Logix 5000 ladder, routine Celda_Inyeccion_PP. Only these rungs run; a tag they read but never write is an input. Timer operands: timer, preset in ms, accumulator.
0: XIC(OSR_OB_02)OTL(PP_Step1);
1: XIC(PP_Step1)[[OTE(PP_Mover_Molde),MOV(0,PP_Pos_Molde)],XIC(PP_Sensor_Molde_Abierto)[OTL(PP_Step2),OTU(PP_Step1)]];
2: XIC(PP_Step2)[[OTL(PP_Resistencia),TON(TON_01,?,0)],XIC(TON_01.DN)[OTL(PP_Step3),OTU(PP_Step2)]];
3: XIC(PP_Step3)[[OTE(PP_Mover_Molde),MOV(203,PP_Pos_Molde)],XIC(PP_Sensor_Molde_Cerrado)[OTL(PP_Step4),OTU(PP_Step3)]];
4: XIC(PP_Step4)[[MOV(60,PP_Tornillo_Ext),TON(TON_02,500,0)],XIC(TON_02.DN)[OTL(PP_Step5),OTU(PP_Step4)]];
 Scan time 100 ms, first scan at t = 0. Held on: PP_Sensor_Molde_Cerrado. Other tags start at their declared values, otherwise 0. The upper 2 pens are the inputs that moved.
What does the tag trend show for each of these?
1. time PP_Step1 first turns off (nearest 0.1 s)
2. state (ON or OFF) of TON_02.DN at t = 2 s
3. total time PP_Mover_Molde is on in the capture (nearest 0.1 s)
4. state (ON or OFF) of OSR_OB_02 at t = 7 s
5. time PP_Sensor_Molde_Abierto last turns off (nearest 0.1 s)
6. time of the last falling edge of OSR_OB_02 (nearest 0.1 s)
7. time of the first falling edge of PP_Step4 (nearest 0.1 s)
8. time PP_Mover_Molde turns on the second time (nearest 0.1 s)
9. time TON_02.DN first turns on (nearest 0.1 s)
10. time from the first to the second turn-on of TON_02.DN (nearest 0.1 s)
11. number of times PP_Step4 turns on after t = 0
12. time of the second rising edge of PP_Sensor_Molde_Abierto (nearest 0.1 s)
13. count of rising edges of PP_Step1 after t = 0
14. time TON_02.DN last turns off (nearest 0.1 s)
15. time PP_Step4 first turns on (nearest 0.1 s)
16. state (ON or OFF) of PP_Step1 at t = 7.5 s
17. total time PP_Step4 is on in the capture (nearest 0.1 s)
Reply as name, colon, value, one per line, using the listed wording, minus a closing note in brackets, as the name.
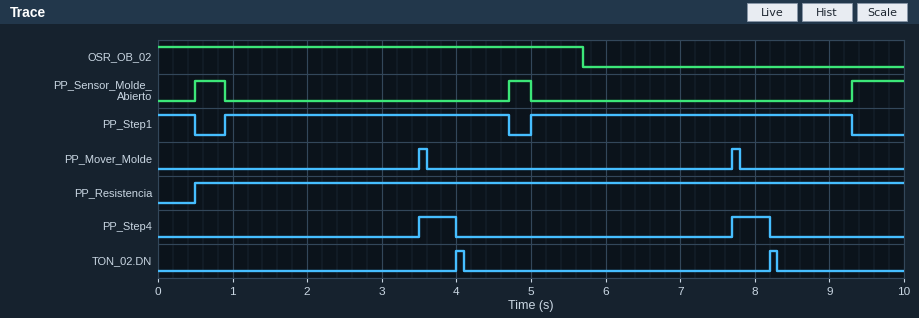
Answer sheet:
time PP_Step1 first turns off: 0.5 s
state (ON or OFF) of TON_02.DN at t = 2 s: OFF
total time PP_Mover_Molde is on in the capture: 0.2 s
state (ON or OFF) of OSR_OB_02 at t = 7 s: OFF
time PP_Sensor_Molde_Abierto last turns off: 5.0 s
time of the last falling edge of OSR_OB_02: 5.7 s
time of the first falling edge of PP_Step4: 4.0 s
time PP_Mover_Molde turns on the second time: 7.7 s
time TON_02.DN first turns on: 4.0 s
time from the first to the second turn-on of TON_02.DN: 4.2 s
number of times PP_Step4 turns on after t = 0: 2
time of the second rising edge of PP_Sensor_Molde_Abierto: 4.7 s
count of rising edges of PP_Step1 after t = 0: 2
time TON_02.DN last turns off: 8.3 s
time PP_Step4 first turns on: 3.5 s
state (ON or OFF) of PP_Step1 at t = 7.5 s: ON
total time PP_Step4 is on in the capture: 1.0 s
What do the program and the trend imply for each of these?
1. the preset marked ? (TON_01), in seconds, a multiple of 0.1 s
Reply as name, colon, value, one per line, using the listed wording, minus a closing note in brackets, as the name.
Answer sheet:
the preset marked ? (TON_01), in seconds, a multiple of 0.1 s: 3.0 s
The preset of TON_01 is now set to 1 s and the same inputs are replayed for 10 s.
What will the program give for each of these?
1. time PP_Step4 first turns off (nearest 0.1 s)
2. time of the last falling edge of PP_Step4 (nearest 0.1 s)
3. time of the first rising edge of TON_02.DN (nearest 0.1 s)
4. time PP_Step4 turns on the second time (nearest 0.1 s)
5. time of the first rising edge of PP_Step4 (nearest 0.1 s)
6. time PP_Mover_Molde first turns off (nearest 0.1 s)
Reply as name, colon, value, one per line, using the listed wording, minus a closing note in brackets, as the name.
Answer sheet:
time PP_Step4 first turns off: 2.0 s
time of the last falling edge of PP_Step4: 6.2 s
time of the first rising edge of TON_02.DN: 2.0 s
time PP_Step4 turns on the second time: 5.7 s
time of the first rising edge of PP_Step4: 1.5 s
time PP_Mover_Molde first turns off: 1.6 s
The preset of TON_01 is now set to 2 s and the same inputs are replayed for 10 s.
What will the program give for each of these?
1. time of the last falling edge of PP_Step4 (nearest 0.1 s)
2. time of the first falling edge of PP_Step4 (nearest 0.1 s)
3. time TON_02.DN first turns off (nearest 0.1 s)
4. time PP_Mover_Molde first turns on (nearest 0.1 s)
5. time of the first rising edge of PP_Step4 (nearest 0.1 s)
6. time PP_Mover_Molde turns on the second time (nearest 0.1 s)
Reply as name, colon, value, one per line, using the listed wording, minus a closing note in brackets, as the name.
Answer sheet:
time of the last falling edge of PP_Step4: 7.2 s
time of the first falling edge of PP_Step4: 3.0 s
time TON_02.DN first turns off: 3.1 s
time PP_Mover_Molde first turns on: 2.5 s
time of the first rising edge of PP_Step4: 2.5 s
time PP_Mover_Molde turns on the second time: 6.7 s
